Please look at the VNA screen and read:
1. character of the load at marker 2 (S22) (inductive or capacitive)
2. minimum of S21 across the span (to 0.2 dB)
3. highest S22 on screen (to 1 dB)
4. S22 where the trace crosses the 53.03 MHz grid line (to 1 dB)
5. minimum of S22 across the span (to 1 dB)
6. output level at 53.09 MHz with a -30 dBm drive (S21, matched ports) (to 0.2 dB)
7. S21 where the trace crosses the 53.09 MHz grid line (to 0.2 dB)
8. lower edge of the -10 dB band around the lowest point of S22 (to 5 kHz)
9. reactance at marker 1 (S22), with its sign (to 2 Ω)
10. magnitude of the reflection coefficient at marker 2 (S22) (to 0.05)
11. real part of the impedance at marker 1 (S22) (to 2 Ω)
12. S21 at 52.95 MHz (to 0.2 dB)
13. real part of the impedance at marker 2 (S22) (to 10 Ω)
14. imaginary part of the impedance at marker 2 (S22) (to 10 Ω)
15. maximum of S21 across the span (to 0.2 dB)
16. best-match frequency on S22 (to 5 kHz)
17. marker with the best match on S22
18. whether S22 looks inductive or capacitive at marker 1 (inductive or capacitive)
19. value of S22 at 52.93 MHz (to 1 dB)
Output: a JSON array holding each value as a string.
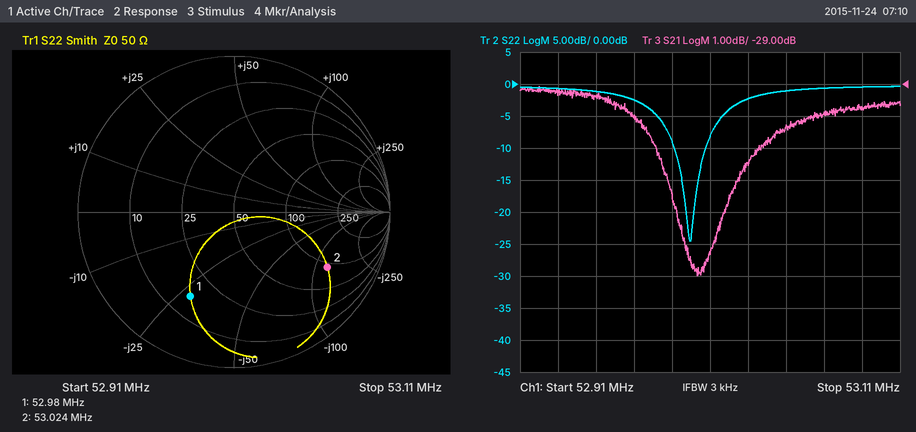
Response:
["capacitive", "-35.0 dB", "0 dB", "-2 dB", "-25 dB", "-59.8 dBm", "-29.8 dB", "52.990 MHz", "-28 Ω", "0.70", "16 Ω", "-29.4 dB", "90 Ω", "-120 Ω", "-29.0 dB", "53.000 MHz", "marker 1", "capacitive", "-1 dB"]
